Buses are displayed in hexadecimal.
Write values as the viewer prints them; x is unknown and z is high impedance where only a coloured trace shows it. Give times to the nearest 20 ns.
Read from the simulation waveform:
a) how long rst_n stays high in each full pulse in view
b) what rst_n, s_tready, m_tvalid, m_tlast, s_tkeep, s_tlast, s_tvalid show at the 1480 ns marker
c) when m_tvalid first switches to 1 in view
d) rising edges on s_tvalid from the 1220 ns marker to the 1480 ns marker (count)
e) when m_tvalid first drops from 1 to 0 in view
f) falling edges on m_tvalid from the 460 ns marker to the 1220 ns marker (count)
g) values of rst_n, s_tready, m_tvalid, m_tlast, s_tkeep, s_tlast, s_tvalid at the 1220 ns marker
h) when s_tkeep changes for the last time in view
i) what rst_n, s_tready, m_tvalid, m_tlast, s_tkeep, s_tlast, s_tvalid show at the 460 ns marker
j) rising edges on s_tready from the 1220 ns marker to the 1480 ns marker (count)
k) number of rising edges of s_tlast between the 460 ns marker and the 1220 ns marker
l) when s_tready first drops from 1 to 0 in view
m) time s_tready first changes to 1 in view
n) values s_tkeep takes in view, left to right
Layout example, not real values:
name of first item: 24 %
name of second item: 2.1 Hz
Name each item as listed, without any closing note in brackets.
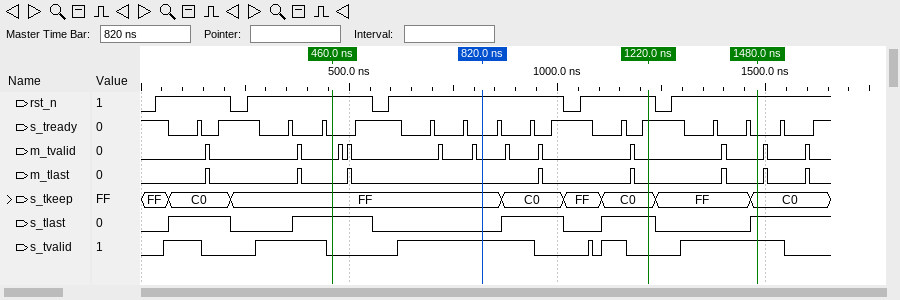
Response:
how long rst_n stays high in each full pulse in view: 180 ns, 300 ns, 420 ns, 180 ns
what rst_n, s_tready, m_tvalid, m_tlast, s_tkeep, s_tlast, s_tvalid show at the 1480 ns marker: rst_n=1, s_tready=0, m_tvalid=0, m_tlast=0, s_tkeep=C0, s_tlast=1, s_tvalid=1
when m_tvalid first switches to 1 in view: 160 ns
rising edges on s_tvalid from the 1220 ns marker to the 1480 ns marker: 1
when m_tvalid first drops from 1 to 0 in view: 160 ns
falling edges on m_tvalid from the 460 ns marker to the 1220 ns marker: 7
values of rst_n, s_tready, m_tvalid, m_tlast, s_tkeep, s_tlast, s_tvalid at the 1220 ns marker: rst_n=1, s_tready=1, m_tvalid=0, m_tlast=0, s_tkeep=C0, s_tlast=1, s_tvalid=0
when s_tkeep changes for the last time in view: 1460 ns
what rst_n, s_tready, m_tvalid, m_tlast, s_tkeep, s_tlast, s_tvalid show at the 460 ns marker: rst_n=1, s_tready=0, m_tvalid=0, m_tlast=0, s_tkeep=FF, s_tlast=1, s_tvalid=0
rising edges on s_tready from the 1220 ns marker to the 1480 ns marker: 2
number of rising edges of s_tlast between the 460 ns marker and the 1220 ns marker: 2
when s_tready first drops from 1 to 0 in view: 60 ns
time s_tready first changes to 1 in view: 140 ns
values s_tkeep takes in view, left to right: FF, C0, FF, C0, FF, C0, FF, C0
